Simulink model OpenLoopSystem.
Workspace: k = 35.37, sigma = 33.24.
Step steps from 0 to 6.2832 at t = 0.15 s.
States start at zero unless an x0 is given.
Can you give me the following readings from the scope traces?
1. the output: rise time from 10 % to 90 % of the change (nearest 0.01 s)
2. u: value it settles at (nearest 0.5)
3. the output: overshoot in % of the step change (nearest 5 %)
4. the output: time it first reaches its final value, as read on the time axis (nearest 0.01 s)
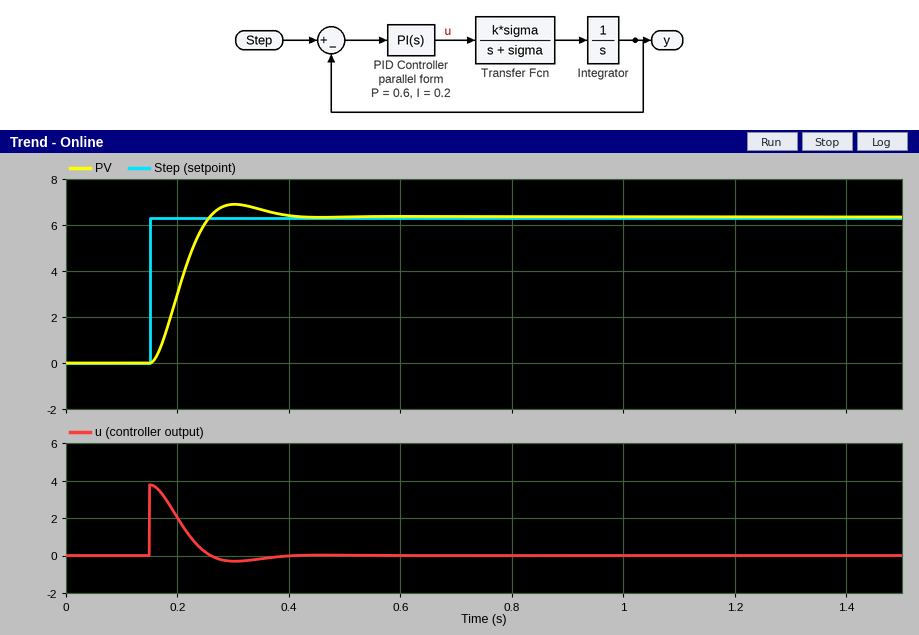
0.07 s
0.0
10 %
0.26 s
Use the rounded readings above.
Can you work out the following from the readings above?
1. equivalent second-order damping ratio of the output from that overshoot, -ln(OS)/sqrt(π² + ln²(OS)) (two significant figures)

0.59
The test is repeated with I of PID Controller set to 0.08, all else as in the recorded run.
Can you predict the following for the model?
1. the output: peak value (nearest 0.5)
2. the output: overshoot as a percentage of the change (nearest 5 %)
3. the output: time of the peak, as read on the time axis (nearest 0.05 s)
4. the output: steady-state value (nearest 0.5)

7.0
10 %
0.30 s
6.5
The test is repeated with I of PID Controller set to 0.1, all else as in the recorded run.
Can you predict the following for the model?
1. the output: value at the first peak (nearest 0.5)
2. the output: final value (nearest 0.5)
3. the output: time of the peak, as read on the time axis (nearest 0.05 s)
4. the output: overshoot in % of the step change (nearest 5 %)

7.0
6.5
0.30 s
10 %
